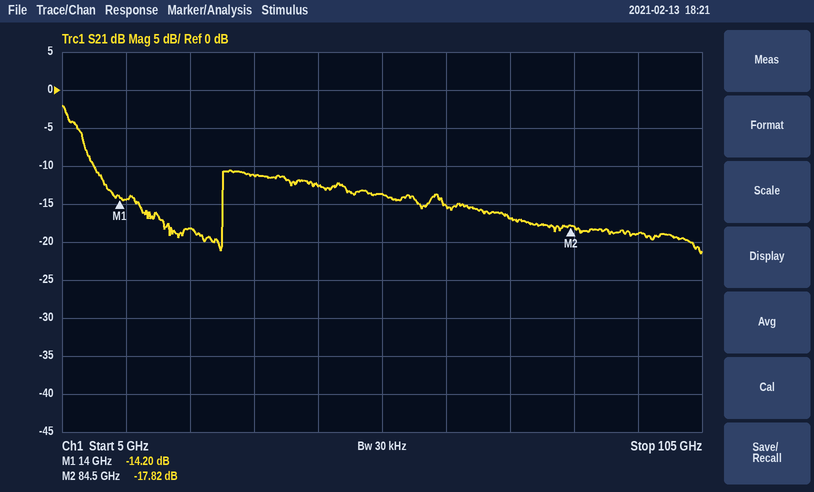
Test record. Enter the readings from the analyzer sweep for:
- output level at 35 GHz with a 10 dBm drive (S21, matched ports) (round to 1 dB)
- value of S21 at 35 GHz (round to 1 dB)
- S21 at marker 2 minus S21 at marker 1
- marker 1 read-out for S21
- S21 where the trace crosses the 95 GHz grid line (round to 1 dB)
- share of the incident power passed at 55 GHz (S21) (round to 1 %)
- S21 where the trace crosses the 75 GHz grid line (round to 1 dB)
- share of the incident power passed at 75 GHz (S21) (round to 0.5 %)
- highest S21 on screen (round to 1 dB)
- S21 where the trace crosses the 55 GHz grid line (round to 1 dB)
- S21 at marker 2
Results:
-1 dBm
-11 dB
-3.62 dB
-14.20 dB
-19 dB
4 %
-17 dB
2.0 %
-2 dB
-14 dB
-17.82 dB
